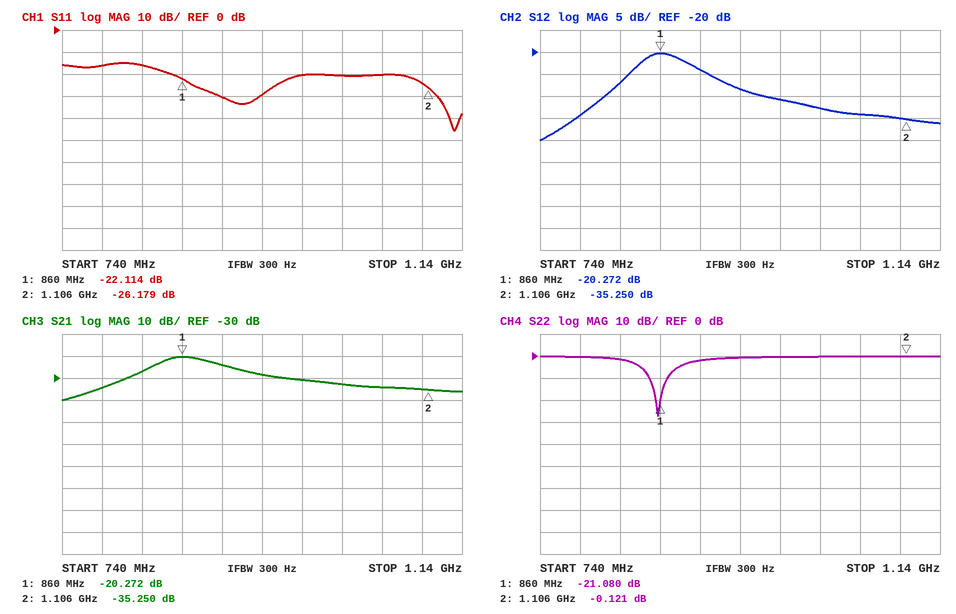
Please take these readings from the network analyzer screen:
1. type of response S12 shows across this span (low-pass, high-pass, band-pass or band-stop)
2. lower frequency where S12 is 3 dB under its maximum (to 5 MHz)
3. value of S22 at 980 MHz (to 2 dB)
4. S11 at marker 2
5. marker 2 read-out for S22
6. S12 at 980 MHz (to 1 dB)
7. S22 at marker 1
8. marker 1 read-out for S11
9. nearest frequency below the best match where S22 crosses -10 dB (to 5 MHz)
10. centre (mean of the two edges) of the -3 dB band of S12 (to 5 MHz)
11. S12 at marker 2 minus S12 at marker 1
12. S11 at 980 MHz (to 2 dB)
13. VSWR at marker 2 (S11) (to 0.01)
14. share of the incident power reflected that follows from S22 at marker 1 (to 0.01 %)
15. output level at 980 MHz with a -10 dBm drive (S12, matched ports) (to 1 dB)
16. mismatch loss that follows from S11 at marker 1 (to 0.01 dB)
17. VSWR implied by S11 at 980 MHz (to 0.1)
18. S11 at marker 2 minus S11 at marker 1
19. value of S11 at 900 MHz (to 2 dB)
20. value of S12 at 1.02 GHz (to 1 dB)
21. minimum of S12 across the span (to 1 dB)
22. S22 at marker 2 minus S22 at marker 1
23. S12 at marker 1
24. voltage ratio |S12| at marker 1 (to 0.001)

band-pass
835 MHz
0 dB
-26.179 dB
-0.121 dB
-31 dB
-21.080 dB
-22.114 dB
850 MHz
865 MHz
-14.978 dB
-20 dB
1.10
0.78 %
-41 dBm
0.03 dB
1.2
-4.065 dB
-30 dB
-33 dB
-40 dB
20.959 dB
-20.272 dB
0.097
